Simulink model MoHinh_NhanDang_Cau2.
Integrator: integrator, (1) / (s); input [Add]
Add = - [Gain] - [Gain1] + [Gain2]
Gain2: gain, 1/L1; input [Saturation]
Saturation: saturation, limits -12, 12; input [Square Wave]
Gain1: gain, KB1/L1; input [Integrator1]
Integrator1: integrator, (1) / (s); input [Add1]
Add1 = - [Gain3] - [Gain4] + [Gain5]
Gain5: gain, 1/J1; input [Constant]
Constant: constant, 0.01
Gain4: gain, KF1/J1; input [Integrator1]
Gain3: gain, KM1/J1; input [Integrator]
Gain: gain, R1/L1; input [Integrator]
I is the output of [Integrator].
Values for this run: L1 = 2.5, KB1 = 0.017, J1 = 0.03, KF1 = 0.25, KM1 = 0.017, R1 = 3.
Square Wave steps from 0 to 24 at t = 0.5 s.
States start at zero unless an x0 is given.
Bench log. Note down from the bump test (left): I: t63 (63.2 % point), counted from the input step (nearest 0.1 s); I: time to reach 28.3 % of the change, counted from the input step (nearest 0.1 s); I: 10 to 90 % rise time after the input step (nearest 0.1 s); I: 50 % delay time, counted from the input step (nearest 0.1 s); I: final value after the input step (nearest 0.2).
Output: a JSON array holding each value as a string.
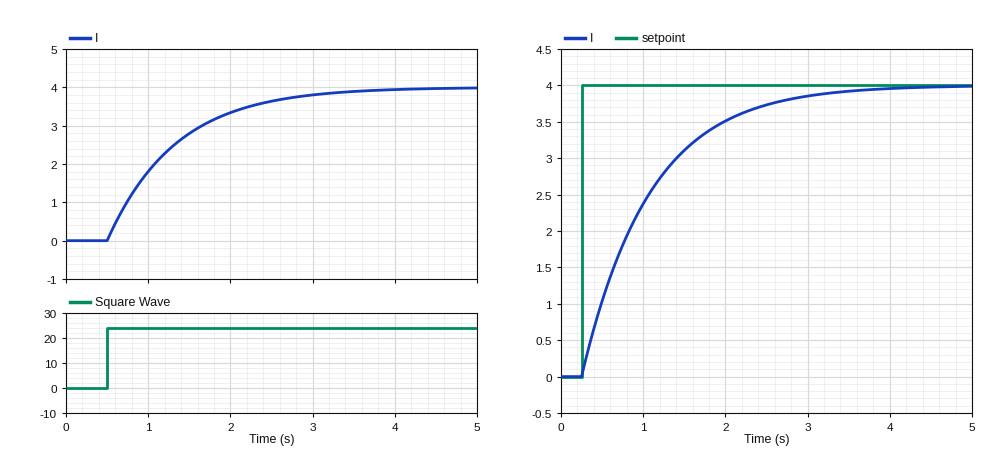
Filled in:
["0.8 s", "0.3 s", "1.8 s", "0.6 s", "4.0"]
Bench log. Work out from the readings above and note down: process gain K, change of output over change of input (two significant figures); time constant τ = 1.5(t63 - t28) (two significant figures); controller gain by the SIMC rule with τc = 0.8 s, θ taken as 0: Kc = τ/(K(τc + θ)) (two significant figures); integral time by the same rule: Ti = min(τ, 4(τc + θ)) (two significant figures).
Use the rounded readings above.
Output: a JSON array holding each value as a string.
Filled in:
["0.17", "0.75 s", "5.5", "0.75 s"]
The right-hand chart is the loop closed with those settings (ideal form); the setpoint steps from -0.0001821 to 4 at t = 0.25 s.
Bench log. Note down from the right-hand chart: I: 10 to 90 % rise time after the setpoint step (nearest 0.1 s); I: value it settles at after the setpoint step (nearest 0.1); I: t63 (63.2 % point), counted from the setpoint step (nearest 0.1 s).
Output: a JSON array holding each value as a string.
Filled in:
["1.8 s", "4.0", "0.8 s"]
